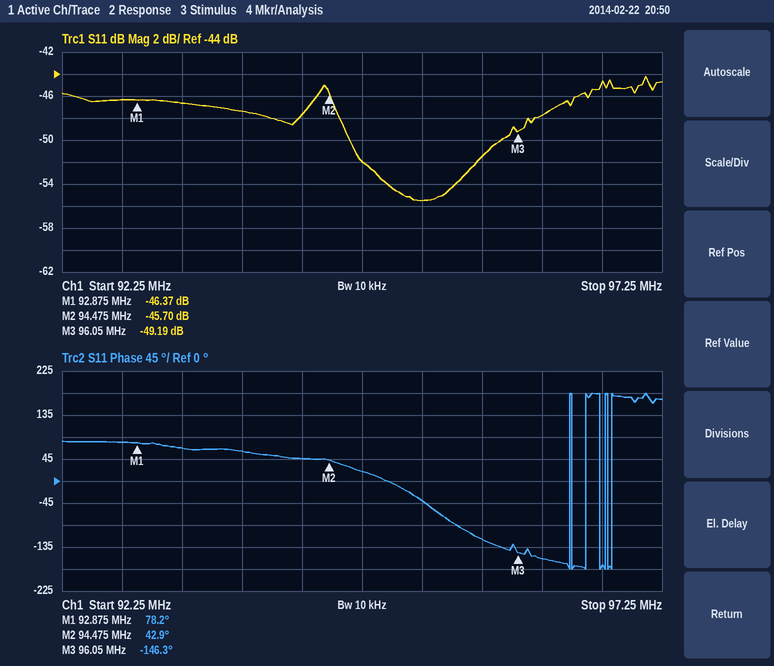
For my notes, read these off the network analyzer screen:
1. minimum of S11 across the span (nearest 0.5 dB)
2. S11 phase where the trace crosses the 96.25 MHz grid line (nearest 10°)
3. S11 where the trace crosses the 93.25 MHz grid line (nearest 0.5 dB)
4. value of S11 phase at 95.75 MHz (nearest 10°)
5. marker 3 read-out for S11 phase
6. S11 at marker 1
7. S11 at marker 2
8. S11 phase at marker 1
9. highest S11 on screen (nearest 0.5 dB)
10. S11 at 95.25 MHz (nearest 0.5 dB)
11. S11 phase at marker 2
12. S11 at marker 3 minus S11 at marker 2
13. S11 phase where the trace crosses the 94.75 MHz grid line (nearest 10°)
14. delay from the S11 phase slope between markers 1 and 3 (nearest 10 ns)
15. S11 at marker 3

-55.5 dB
-160°
-46.5 dB
-120°
-146.3°
-46.37 dB
-45.70 dB
78.2°
-44.0 dB
-55.5 dB
42.9°
-3.49 dB
20°
200 ns
-49.19 dB
